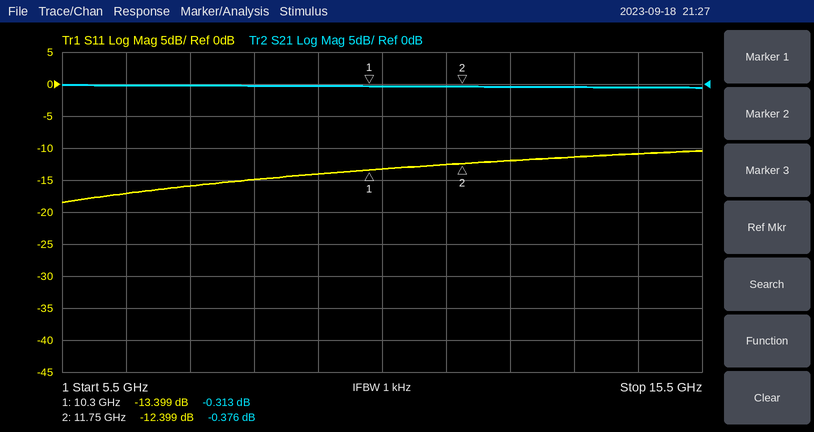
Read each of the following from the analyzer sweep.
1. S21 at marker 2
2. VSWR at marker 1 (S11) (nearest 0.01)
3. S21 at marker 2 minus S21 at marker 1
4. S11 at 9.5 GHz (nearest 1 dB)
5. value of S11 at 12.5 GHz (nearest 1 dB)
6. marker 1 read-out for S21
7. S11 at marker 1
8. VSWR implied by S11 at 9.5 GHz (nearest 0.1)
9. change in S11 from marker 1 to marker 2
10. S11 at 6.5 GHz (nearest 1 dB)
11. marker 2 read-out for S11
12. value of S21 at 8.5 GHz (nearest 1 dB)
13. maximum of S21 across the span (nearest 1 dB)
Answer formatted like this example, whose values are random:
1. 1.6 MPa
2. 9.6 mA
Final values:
1. -0.376 dB
2. 1.54
3. -0.063 dB
4. -14 dB
5. -12 dB
6. -0.313 dB
7. -13.399 dB
8. 1.5
9. 1.000 dB
10. -17 dB
11. -12.399 dB
12. 0 dB
13. 0 dB
